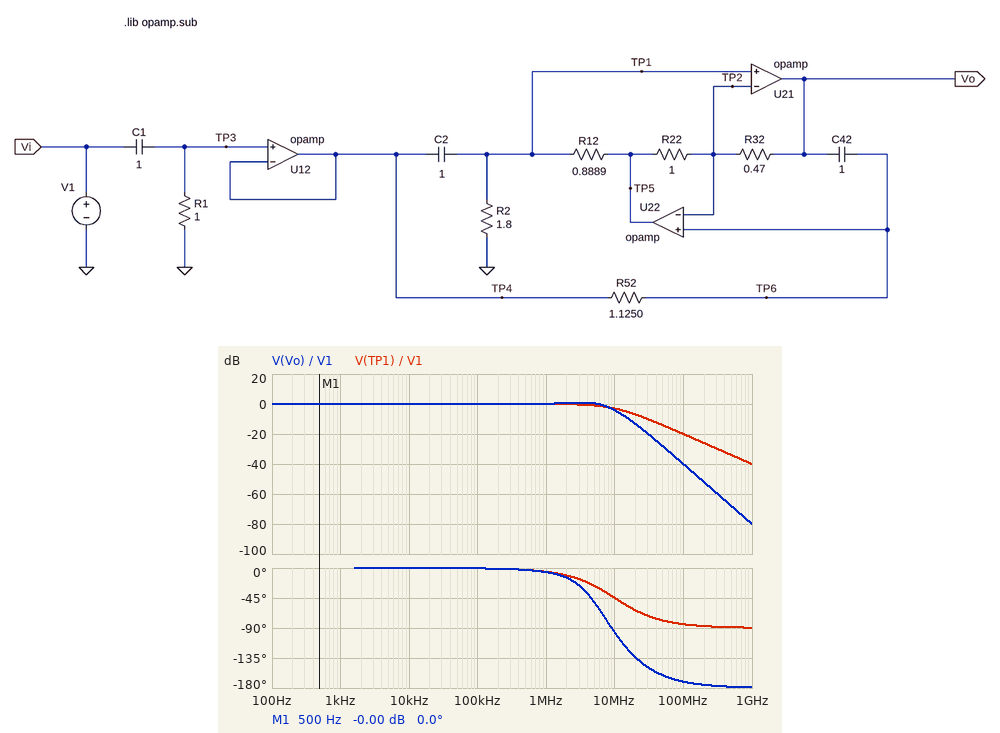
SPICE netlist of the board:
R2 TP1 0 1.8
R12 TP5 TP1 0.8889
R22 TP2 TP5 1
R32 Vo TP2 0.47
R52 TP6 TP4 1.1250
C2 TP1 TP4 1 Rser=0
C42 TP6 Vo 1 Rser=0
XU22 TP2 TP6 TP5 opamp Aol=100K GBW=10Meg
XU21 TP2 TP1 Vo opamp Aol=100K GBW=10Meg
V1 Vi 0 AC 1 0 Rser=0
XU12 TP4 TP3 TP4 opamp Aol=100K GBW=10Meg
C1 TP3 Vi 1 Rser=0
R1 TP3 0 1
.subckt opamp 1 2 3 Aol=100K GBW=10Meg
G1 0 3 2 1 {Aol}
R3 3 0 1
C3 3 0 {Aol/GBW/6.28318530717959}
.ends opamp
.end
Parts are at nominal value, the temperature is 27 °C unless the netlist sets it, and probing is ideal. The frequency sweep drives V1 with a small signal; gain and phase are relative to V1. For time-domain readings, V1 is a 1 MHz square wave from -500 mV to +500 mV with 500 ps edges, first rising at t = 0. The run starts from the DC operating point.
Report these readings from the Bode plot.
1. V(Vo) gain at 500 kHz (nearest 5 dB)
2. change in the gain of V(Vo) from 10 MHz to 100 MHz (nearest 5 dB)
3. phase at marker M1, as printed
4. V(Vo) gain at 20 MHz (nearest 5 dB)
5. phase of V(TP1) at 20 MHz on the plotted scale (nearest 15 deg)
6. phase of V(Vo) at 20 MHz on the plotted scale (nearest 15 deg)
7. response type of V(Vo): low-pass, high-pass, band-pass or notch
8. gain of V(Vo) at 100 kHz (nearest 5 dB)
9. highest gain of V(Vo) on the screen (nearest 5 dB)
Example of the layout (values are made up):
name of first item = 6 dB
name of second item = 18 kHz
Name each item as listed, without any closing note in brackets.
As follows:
V(Vo) gain at 500 kHz = 0 dB
change in the gain of V(Vo) from 10 MHz to 100 MHz = -35 dB
phase at marker M1, as printed = 0.0 deg
V(Vo) gain at 20 MHz = -15 dB
phase of V(TP1) at 20 MHz on the plotted scale = -60 deg
phase of V(Vo) at 20 MHz on the plotted scale = -135 deg
response type of V(Vo): low-pass, high-pass, band-pass or notch = low-pass
gain of V(Vo) at 100 kHz = 0 dB
highest gain of V(Vo) on the screen = 0 dB
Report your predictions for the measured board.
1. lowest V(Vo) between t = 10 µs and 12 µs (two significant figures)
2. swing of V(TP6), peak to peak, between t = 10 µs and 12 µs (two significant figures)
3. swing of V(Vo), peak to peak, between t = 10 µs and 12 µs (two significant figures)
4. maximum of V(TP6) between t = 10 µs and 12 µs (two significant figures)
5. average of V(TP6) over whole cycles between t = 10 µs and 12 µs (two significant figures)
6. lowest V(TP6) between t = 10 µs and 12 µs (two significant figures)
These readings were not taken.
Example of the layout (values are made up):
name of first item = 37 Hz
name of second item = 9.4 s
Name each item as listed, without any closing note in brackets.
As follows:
lowest V(Vo) between t = 10 µs and 12 µs = -120 mV
swing of V(TP6), peak to peak, between t = 10 µs and 12 µs = 1.2 V
swing of V(Vo), peak to peak, between t = 10 µs and 12 µs = 1.2 V
maximum of V(TP6) between t = 10 µs and 12 µs = 1.1 V
average of V(TP6) over whole cycles between t = 10 µs and 12 µs = 500 mV
lowest V(TP6) between t = 10 µs and 12 µs = -120 mV
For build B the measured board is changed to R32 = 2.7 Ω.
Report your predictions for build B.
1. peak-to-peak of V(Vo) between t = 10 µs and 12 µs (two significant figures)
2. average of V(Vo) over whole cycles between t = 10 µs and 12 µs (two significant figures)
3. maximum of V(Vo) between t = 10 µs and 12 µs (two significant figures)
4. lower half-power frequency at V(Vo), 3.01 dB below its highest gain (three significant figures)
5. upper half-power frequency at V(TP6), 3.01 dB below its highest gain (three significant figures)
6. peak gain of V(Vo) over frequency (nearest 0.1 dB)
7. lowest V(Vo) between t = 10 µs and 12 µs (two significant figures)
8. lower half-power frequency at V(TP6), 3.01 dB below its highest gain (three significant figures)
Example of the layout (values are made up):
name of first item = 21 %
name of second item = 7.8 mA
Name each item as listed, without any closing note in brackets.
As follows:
peak-to-peak of V(Vo) between t = 10 µs and 12 µs = 1.3 V
average of V(Vo) over whole cycles between t = 10 µs and 12 µs = 500 mV
maximum of V(Vo) between t = 10 µs and 12 µs = 1.2 V
lower half-power frequency at V(Vo), 3.01 dB below its highest gain = 103 mHz
upper half-power frequency at V(TP6), 3.01 dB below its highest gain = 10.3 MHz
peak gain of V(Vo) over frequency = 1.2 dB
lowest V(Vo) between t = 10 µs and 12 µs = -160 mV
lower half-power frequency at V(TP6), 3.01 dB below its highest gain = 276 mHz
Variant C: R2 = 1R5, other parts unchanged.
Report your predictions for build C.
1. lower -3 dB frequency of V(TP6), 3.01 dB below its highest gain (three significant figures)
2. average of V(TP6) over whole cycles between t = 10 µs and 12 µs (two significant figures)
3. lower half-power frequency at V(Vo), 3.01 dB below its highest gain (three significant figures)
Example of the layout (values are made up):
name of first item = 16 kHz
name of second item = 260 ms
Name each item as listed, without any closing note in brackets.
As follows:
lower -3 dB frequency of V(TP6), 3.01 dB below its highest gain = 343 mHz
average of V(TP6) over whole cycles between t = 10 µs and 12 µs = 500 mV
lower half-power frequency at V(Vo), 3.01 dB below its highest gain = 259 mHz
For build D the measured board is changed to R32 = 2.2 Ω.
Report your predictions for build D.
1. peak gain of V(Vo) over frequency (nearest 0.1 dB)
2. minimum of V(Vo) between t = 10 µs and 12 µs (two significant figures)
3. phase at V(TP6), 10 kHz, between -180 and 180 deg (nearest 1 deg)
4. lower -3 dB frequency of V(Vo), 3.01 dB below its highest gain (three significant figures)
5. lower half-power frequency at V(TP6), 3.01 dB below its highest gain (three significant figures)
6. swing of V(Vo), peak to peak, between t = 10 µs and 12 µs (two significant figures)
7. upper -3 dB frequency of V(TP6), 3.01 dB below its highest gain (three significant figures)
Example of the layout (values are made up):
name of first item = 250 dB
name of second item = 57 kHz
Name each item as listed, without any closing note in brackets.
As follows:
peak gain of V(Vo) over frequency = 1.2 dB
minimum of V(Vo) between t = 10 µs and 12 µs = -160 mV
phase at V(TP6), 10 kHz, between -180 and 180 deg = 0 deg
lower -3 dB frequency of V(Vo), 3.01 dB below its highest gain = 116 mHz
lower half-power frequency at V(TP6), 3.01 dB below its highest gain = 278 mHz
swing of V(Vo), peak to peak, between t = 10 µs and 12 µs = 1.3 V
upper -3 dB frequency of V(TP6), 3.01 dB below its highest gain = 10.1 MHz
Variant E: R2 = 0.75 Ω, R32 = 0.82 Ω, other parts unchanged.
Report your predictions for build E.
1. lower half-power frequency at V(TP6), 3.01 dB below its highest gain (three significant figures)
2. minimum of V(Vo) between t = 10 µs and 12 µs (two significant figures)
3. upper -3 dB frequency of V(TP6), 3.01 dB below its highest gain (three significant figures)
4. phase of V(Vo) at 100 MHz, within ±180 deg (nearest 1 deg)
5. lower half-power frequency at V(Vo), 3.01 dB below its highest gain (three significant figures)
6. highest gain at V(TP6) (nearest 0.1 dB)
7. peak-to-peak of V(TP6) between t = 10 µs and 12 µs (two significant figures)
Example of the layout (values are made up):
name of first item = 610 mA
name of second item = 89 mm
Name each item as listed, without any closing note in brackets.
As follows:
lower half-power frequency at V(TP6), 3.01 dB below its highest gain = 423 mHz
minimum of V(Vo) between t = 10 µs and 12 µs = -140 mV
upper -3 dB frequency of V(TP6), 3.01 dB below its highest gain = 8.71 MHz
phase of V(Vo) at 100 MHz, within ±180 deg = -171 deg
lower half-power frequency at V(Vo), 3.01 dB below its highest gain = 231 mHz
highest gain at V(TP6) = 1.1 dB
peak-to-peak of V(TP6) between t = 10 µs and 12 µs = 1.3 V
